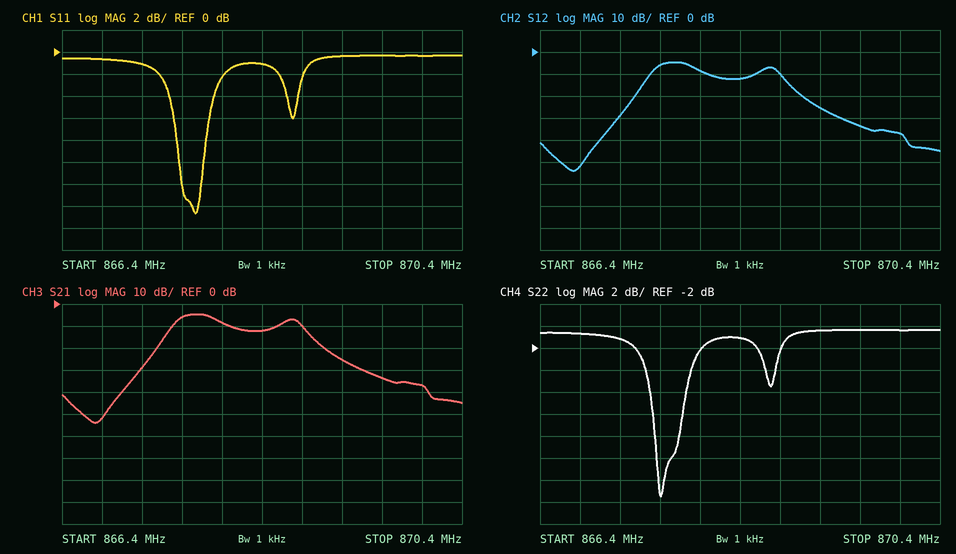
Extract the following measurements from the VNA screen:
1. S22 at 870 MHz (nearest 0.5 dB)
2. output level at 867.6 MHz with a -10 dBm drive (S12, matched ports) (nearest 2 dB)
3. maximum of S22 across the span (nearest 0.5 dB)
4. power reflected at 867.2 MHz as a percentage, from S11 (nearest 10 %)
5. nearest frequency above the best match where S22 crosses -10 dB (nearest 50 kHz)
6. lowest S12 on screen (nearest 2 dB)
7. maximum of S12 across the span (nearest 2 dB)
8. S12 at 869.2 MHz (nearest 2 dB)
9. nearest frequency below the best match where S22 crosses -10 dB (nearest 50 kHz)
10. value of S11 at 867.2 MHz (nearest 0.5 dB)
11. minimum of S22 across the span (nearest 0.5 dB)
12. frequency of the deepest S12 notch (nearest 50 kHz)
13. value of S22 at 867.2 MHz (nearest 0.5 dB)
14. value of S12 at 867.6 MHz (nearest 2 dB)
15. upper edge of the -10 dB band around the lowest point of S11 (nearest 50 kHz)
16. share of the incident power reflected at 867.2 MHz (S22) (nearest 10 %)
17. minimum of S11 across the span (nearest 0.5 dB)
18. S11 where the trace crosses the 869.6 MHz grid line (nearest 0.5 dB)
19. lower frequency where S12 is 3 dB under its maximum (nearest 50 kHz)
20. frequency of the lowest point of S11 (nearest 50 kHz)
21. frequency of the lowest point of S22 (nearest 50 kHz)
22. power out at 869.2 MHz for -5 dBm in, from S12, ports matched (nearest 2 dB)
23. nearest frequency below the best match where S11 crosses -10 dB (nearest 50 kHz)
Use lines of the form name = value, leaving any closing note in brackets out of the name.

S22 at 870 MHz = -0.5 dB
output level at 867.6 MHz with a -10 dBm drive (S12, matched ports) = -16 dBm
maximum of S22 across the span = -0.5 dB
power reflected at 867.2 MHz as a percentage, from S11 = 80 %
nearest frequency above the best match where S22 crosses -10 dB = 867.80 MHz
lowest S12 on screen = -54 dB
maximum of S12 across the span = -4 dB
S12 at 869.2 MHz = -26 dB
nearest frequency below the best match where S22 crosses -10 dB = 867.55 MHz
value of S11 at 867.2 MHz = -1.0 dB
minimum of S22 across the span = -15.5 dB
frequency of the deepest S12 notch = 866.75 MHz
value of S22 at 867.2 MHz = -1.0 dB
value of S12 at 867.6 MHz = -6 dB
upper edge of the -10 dB band around the lowest point of S11 = 867.80 MHz
share of the incident power reflected at 867.2 MHz (S22) = 80 %
minimum of S11 across the span = -14.5 dB
S11 where the trace crosses the 869.6 MHz grid line = -0.5 dB
lower frequency where S12 is 3 dB under its maximum = 867.55 MHz
frequency of the lowest point of S11 = 867.75 MHz
frequency of the lowest point of S22 = 867.60 MHz
power out at 869.2 MHz for -5 dBm in, from S12, ports matched = -30 dBm
nearest frequency below the best match where S11 crosses -10 dB = 867.55 MHz
